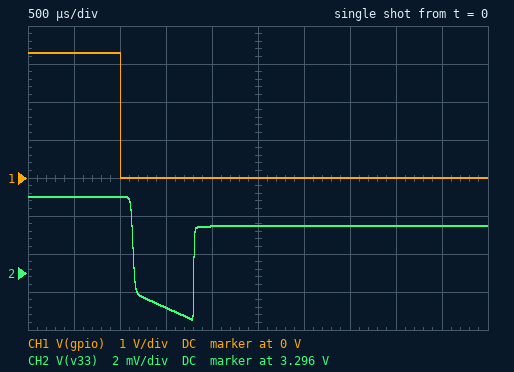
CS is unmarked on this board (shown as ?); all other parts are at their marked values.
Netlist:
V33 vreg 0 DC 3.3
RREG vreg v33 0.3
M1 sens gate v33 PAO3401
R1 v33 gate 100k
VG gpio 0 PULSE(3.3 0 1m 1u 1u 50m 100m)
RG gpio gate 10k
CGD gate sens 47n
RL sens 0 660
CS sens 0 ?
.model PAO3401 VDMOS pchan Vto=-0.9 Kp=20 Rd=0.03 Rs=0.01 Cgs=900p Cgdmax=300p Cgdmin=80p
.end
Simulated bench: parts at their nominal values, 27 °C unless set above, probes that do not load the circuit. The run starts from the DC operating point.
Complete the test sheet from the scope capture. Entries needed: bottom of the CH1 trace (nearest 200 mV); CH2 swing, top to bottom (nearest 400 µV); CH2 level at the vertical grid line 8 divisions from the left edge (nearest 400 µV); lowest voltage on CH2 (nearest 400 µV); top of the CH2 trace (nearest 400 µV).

0 V
6.4 mV
3.2984 V
3.2936 V
3.3000 V
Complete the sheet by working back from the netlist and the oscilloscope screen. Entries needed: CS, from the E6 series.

3.3 µF
